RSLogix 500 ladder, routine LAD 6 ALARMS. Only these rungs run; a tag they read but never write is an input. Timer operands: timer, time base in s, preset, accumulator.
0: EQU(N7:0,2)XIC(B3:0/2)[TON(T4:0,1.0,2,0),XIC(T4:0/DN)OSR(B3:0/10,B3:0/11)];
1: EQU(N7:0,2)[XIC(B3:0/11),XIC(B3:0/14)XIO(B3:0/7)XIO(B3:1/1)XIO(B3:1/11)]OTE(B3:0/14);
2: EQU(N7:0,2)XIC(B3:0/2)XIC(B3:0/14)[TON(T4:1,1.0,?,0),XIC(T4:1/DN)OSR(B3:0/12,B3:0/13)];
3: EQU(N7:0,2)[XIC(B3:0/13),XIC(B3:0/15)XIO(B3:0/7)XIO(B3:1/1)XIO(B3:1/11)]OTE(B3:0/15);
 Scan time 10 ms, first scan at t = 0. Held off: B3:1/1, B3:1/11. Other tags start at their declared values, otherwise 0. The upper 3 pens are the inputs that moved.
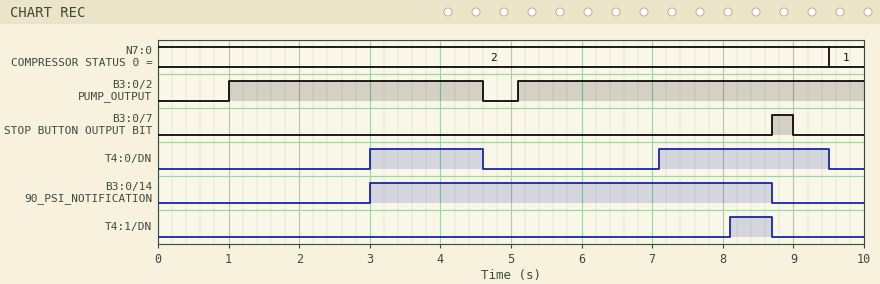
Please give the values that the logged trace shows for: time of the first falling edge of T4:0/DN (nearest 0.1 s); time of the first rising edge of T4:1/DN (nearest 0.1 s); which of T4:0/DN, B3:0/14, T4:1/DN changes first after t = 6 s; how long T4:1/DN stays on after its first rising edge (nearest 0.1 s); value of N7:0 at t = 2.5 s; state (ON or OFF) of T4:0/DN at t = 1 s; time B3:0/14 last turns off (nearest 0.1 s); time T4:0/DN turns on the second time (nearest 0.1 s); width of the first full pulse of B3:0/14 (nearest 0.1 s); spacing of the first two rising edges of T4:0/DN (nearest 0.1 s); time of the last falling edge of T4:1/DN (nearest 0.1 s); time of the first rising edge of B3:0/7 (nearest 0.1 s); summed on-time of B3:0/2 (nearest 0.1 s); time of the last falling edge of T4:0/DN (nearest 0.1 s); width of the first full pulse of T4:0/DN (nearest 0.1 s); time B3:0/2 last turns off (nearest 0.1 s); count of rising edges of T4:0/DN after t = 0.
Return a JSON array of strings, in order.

["4.6 s", "8.1 s", "T4:0/DN", "0.6 s", "2", "OFF", "8.7 s", "7.1 s", "5.7 s", "4.1 s", "8.7 s", "8.7 s", "8.5 s", "9.5 s", "1.6 s", "4.6 s", "2"]
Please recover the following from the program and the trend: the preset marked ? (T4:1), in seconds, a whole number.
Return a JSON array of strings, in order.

["3 s"]
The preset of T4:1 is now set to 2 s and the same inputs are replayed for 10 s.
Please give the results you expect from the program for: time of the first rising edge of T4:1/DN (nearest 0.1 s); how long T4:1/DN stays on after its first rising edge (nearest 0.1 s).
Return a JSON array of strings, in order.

["7.1 s", "1.6 s"]
